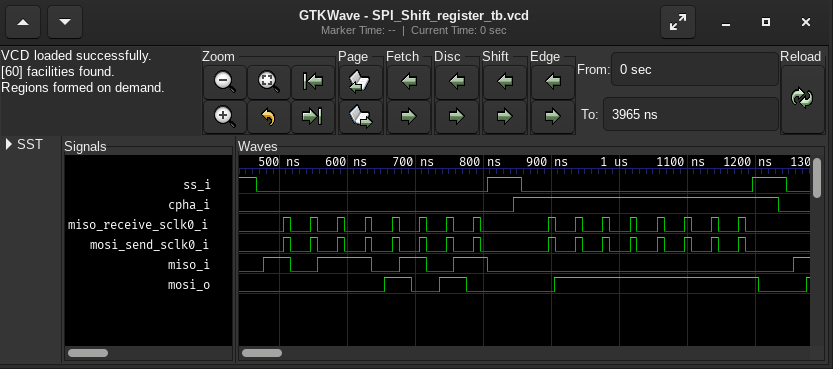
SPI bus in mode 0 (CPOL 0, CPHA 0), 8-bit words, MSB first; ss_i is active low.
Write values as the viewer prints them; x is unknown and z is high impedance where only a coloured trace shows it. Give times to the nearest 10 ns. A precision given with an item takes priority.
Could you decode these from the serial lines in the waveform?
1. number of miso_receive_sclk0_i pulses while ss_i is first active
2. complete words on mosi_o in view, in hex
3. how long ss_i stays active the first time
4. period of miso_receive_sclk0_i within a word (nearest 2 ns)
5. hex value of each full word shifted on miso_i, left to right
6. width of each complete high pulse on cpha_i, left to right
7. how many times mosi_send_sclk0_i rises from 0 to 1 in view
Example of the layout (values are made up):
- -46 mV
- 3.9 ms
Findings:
- 8
- 0A, 7F
- 340 ns
- 40 ns
- B5, 00
- 390 ns
- 16
